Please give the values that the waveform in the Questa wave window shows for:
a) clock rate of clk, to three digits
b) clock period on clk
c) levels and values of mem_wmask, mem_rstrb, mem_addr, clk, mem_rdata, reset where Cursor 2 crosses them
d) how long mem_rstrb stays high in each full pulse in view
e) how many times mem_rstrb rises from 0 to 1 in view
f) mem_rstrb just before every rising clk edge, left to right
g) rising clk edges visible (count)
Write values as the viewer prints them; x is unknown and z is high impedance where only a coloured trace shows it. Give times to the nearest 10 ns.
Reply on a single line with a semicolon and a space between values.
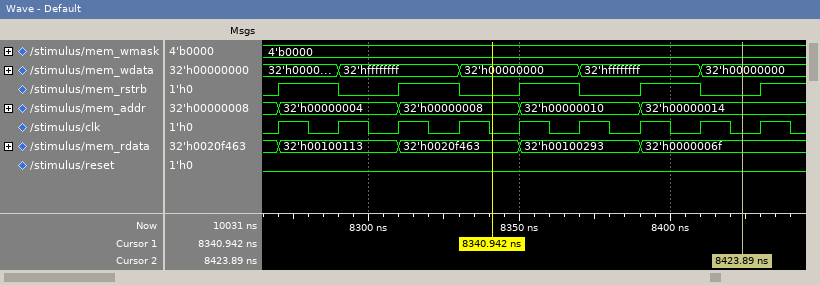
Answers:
50.0 MHz; 20 ns; mem_wmask=4'b0000, mem_rstrb=0, mem_addr=32'h00000014, clk=0, mem_rdata=32'h0000006f, reset=0; 20 ns, 20 ns, 20 ns, 20 ns; 5; 0 1 0 1 0 1 0 1 0; 9
